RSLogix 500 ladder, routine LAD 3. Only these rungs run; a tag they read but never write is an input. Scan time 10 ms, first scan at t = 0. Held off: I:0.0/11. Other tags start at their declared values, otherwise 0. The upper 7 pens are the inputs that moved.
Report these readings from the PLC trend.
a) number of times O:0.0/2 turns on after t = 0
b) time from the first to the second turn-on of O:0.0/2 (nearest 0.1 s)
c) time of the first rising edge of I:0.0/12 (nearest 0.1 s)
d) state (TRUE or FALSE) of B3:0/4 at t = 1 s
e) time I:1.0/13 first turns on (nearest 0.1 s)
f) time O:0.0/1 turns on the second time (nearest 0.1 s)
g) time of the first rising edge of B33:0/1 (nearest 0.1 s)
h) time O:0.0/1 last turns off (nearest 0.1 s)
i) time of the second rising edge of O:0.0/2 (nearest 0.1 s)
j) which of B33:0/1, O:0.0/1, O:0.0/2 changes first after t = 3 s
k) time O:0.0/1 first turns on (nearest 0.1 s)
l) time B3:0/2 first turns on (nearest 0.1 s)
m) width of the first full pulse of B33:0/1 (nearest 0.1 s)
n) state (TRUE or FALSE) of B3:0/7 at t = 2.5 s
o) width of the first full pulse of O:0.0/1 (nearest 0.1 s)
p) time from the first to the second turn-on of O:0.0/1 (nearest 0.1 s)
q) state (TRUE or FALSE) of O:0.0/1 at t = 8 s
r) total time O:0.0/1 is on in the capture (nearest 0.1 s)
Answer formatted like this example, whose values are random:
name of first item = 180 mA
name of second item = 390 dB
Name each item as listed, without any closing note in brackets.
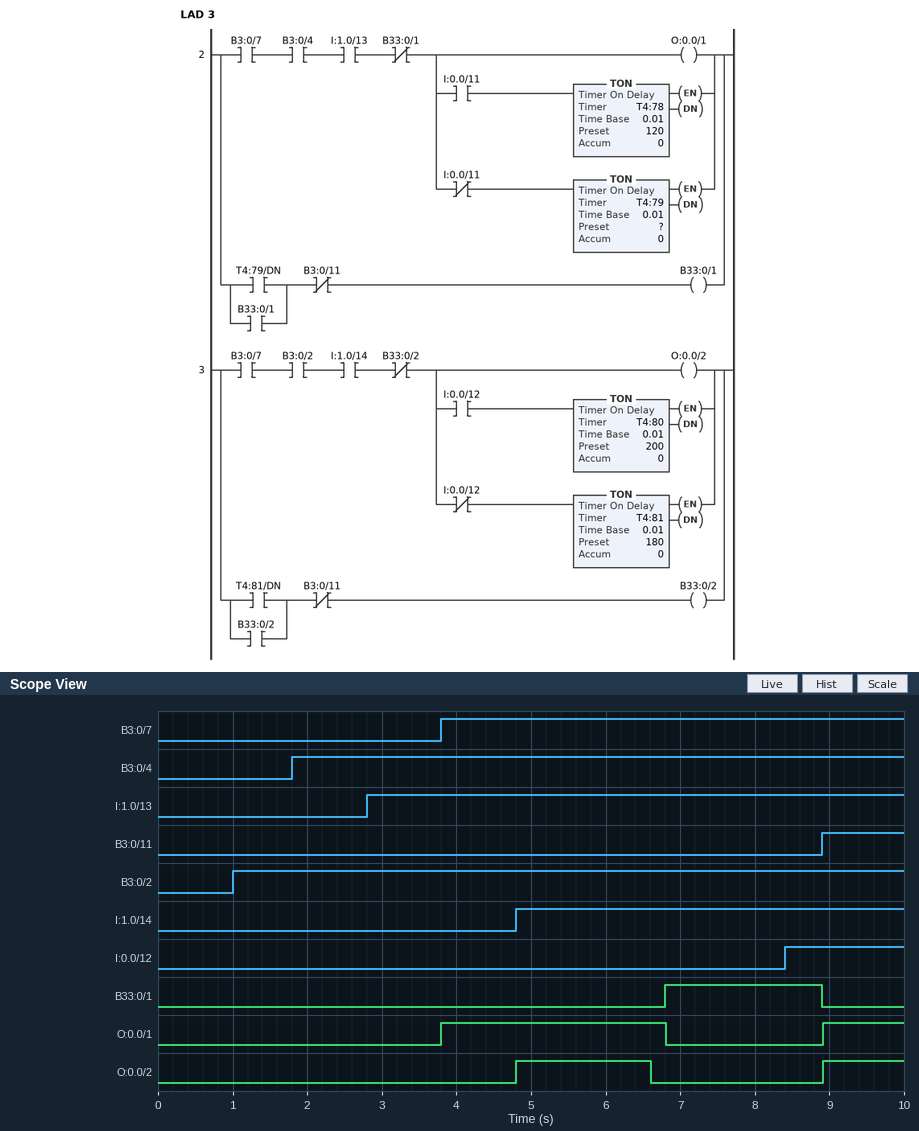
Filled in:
number of times O:0.0/2 turns on after t = 0 = 2
time from the first to the second turn-on of O:0.0/2 = 4.1 s
time of the first rising edge of I:0.0/12 = 8.4 s
state (TRUE or FALSE) of B3:0/4 at t = 1 s = FALSE
time I:1.0/13 first turns on = 2.8 s
time O:0.0/1 turns on the second time = 8.9 s
time of the first rising edge of B33:0/1 = 6.8 s
time O:0.0/1 last turns off = 6.8 s
time of the second rising edge of O:0.0/2 = 8.9 s
which of B33:0/1, O:0.0/1, O:0.0/2 changes first after t = 3 s = O:0.0/1
time O:0.0/1 first turns on = 3.8 s
time B3:0/2 first turns on = 1.0 s
width of the first full pulse of B33:0/1 = 2.1 s
state (TRUE or FALSE) of B3:0/7 at t = 2.5 s = FALSE
width of the first full pulse of O:0.0/1 = 3.0 s
time from the first to the second turn-on of O:0.0/1 = 5.1 s
state (TRUE or FALSE) of O:0.0/1 at t = 8 s = FALSE
total time O:0.0/1 is on in the capture = 4.1 s
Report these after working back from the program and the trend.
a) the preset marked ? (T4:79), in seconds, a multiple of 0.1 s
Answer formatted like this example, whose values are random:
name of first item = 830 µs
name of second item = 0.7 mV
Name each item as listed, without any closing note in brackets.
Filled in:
the preset marked ? (T4:79), in seconds, a multiple of 0.1 s = 3.0 s
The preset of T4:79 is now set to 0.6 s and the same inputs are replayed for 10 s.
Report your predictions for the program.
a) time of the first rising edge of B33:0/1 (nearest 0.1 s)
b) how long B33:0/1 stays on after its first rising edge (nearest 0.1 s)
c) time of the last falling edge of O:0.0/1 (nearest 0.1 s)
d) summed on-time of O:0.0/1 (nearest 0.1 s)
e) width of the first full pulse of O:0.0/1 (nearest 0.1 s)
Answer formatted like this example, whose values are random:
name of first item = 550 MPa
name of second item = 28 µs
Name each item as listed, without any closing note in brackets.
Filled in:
time of the first rising edge of B33:0/1 = 4.4 s
how long B33:0/1 stays on after its first rising edge = 4.5 s
time of the last falling edge of O:0.0/1 = 4.4 s
summed on-time of O:0.0/1 = 1.7 s
width of the first full pulse of O:0.0/1 = 0.6 s
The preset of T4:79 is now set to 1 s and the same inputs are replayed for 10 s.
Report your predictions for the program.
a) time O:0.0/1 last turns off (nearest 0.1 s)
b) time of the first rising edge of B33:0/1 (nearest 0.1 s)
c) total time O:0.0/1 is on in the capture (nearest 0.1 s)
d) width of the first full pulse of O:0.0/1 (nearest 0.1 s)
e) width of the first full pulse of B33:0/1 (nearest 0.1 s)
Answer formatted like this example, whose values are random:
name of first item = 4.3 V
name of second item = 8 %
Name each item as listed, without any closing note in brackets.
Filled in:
time O:0.0/1 last turns off = 4.8 s
time of the first rising edge of B33:0/1 = 4.8 s
total time O:0.0/1 is on in the capture = 2.1 s
width of the first full pulse of O:0.0/1 = 1.0 s
width of the first full pulse of B33:0/1 = 4.1 s
